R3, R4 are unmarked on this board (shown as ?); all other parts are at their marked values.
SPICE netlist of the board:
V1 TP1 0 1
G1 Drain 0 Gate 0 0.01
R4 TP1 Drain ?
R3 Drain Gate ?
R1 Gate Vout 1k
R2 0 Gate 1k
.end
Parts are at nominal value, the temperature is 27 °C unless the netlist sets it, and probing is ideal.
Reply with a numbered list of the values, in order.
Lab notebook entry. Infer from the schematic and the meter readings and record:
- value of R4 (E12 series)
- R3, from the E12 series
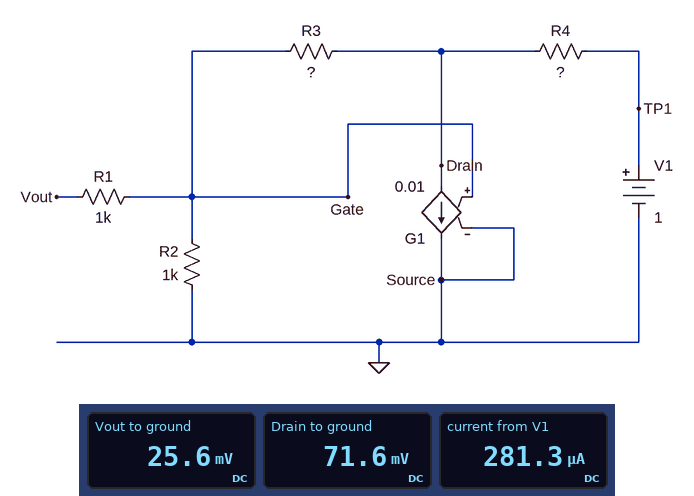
1. 3.3 kΩ
2. 1.8 kΩ
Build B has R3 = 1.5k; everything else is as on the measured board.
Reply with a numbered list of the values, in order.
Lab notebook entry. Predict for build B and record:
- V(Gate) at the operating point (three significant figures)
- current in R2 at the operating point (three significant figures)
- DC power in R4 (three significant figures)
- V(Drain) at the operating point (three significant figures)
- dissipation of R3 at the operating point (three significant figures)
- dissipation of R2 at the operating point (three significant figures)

1. 25.8 mV
2. 25.8 µA
3. 265 µW
4. 64.4 mV
5. 996 nW
6. 664 nW
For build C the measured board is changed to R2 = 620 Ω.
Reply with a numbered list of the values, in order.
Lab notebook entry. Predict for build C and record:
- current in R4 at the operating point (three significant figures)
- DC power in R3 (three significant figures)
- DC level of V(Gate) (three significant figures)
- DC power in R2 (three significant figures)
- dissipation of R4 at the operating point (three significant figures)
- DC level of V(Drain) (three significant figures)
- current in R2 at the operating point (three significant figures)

1. 275 µA
2. 2.63 µW
3. 23.7 mV
4. 905 nW
5. 250 µW
6. 92.4 mV
7. 38.2 µA
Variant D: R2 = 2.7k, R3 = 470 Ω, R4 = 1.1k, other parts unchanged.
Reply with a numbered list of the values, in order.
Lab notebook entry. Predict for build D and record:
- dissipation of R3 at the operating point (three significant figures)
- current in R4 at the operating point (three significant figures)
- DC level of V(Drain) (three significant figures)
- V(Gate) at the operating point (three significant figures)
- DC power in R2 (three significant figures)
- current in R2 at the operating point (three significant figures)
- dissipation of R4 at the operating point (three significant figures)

1. 407 nW
2. 824 µA
3. 93.3 mV
4. 79.5 mV
5. 2.34 µW
6. 29.4 µA
7. 747 µW
